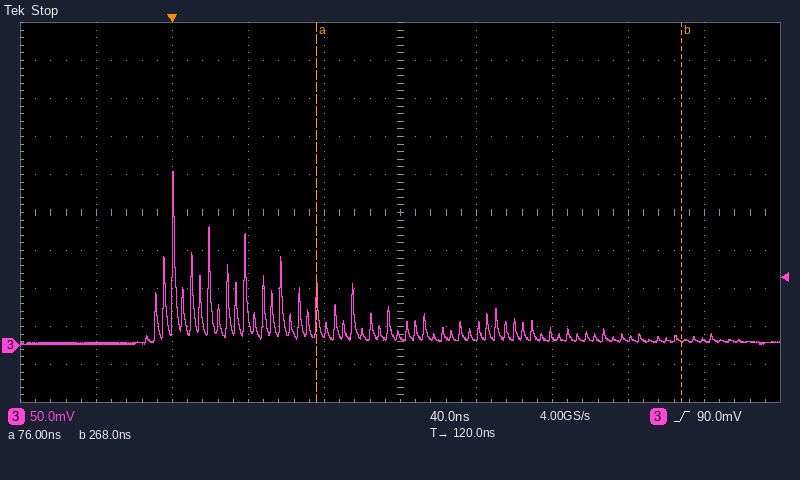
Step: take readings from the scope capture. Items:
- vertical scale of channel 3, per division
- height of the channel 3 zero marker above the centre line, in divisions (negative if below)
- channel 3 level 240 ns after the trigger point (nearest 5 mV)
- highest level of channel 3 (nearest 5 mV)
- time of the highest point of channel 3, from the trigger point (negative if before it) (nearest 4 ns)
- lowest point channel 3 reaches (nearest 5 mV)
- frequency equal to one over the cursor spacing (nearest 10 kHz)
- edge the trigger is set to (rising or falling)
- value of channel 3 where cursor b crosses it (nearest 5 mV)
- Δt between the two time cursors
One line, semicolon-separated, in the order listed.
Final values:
50 mV; -3.5 div; 10 mV; 230 mV; 0 ns; 0 mV; 5.21 MHz; rising; 5 mV; 192 ns
